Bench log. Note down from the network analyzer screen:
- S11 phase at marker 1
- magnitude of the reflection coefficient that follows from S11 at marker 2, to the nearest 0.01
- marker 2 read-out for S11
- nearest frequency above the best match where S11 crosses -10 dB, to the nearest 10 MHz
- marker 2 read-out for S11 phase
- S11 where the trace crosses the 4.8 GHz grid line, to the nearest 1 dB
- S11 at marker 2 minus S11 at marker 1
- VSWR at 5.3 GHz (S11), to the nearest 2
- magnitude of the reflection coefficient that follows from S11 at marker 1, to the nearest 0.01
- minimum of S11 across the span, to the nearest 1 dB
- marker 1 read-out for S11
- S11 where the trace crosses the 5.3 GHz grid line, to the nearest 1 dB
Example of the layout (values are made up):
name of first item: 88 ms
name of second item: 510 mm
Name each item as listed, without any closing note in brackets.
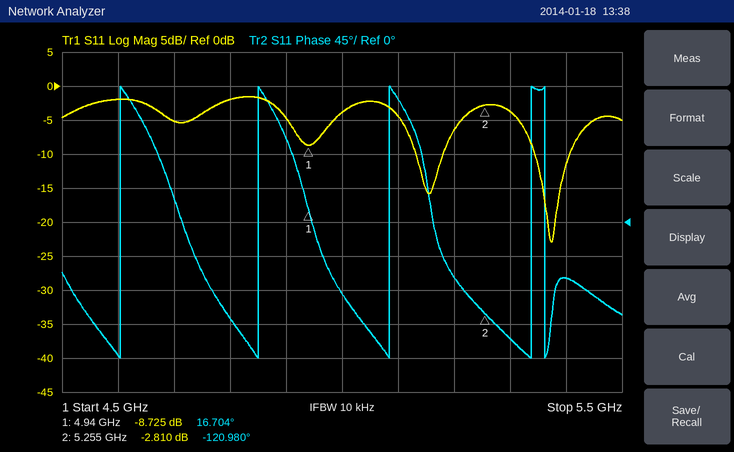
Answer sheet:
S11 phase at marker 1: 16.704°
magnitude of the reflection coefficient that follows from S11 at marker 2, to the nearest 0.01: 0.72
marker 2 read-out for S11: -2.810 dB
nearest frequency above the best match where S11 crosses -10 dB, to the nearest 10 MHz: 5.41 GHz
marker 2 read-out for S11 phase: -120.980°
S11 where the trace crosses the 4.8 GHz grid line, to the nearest 1 dB: -2 dB
S11 at marker 2 minus S11 at marker 1: 5.915 dB
VSWR at 5.3 GHz (S11), to the nearest 2: 4
magnitude of the reflection coefficient that follows from S11 at marker 1, to the nearest 0.01: 0.37
minimum of S11 across the span, to the nearest 1 dB: -23 dB
marker 1 read-out for S11: -8.725 dB
S11 where the trace crosses the 5.3 GHz grid line, to the nearest 1 dB: -4 dB
